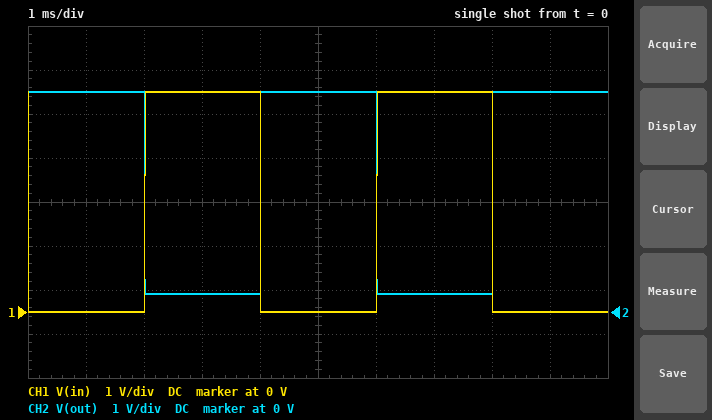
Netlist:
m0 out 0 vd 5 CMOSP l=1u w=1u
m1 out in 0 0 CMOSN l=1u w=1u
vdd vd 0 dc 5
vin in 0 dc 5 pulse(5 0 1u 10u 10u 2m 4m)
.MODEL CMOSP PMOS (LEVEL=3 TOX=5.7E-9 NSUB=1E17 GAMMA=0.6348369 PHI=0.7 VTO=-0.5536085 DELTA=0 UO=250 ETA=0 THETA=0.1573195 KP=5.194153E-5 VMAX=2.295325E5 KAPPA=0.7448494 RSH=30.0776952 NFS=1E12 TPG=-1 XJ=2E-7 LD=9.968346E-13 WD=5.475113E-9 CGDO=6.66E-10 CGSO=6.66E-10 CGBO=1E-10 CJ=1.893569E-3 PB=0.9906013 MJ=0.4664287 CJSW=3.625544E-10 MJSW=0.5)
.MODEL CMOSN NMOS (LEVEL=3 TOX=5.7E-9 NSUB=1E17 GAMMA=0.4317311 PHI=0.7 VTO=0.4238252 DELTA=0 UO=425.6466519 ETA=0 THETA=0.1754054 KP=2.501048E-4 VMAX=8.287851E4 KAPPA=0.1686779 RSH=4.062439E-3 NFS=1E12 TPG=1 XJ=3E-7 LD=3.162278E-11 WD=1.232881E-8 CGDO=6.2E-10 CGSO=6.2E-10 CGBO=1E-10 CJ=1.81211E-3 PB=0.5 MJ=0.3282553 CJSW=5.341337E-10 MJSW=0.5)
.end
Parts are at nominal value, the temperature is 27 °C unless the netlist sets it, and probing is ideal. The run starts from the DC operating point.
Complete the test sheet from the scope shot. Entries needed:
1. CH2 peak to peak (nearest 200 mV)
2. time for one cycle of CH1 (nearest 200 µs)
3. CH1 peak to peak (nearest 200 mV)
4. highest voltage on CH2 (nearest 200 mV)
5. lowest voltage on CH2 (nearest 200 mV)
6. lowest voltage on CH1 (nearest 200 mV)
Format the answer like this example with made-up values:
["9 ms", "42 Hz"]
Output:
["4.6 V", "4.0 ms", "5.0 V", "5.0 V", "400 mV", "0 V"]
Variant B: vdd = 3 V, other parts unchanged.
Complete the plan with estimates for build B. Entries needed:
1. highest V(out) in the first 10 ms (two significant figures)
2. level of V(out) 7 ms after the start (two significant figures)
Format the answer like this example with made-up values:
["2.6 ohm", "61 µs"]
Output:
["3.0 V", "150 mV"]
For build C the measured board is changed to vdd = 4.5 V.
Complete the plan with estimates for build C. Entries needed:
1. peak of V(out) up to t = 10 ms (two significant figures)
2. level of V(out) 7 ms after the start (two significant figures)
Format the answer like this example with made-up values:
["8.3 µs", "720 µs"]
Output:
["4.5 V", "330 mV"]
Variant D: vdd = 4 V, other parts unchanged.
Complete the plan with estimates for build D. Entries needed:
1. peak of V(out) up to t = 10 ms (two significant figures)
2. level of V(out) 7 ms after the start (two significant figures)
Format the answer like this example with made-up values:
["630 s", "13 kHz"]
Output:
["4.0 V", "260 mV"]
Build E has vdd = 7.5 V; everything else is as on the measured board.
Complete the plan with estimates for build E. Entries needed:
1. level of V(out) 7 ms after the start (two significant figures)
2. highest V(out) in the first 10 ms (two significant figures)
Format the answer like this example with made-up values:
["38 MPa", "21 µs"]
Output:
["900 mV", "7.5 V"]
